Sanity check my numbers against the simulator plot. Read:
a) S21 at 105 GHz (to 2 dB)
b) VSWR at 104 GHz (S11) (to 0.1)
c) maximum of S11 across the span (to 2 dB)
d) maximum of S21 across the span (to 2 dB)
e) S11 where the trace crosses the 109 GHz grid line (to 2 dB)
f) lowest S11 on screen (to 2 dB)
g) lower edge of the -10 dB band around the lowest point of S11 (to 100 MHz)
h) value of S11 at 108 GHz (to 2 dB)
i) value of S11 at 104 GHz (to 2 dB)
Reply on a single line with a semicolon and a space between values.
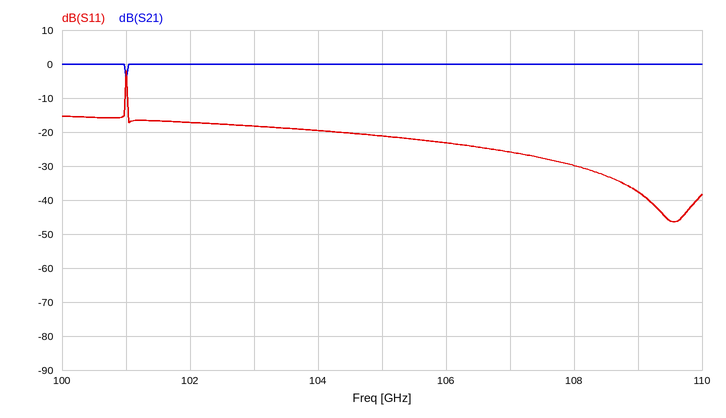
0 dB; 1.2; -2 dB; 0 dB; -38 dB; -46 dB; 101.0 GHz; -30 dB; -20 dB
